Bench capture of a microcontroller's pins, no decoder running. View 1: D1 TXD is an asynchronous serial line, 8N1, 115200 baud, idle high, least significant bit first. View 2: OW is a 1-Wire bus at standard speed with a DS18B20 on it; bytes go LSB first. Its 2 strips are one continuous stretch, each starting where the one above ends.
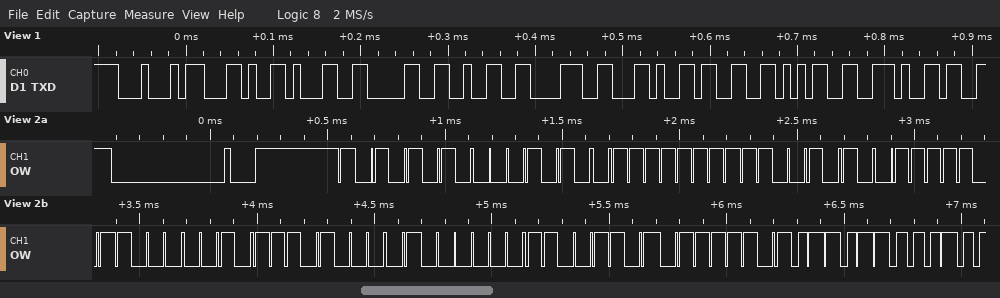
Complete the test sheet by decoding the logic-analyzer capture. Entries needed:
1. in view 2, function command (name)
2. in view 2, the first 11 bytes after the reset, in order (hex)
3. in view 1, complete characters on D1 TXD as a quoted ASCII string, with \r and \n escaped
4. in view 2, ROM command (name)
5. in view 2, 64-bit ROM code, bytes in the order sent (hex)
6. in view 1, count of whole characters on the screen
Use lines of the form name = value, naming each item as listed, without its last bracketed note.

in view 2, function command = Read Scratchpad
in view 2, the first 11 bytes after the reset, in order = 55 28 FF 53 BE 41 17 02 B3 BE 36
in view 1, complete characters on D1 TXD as a quoted ASCII string, with \r and \n escaped = "D,1028,35."
in view 2, ROM command = Match ROM
in view 2, 64-bit ROM code, bytes in the order sent = 28 FF 53 BE 41 17 02 B3
in view 1, count of whole characters on the screen = 10
